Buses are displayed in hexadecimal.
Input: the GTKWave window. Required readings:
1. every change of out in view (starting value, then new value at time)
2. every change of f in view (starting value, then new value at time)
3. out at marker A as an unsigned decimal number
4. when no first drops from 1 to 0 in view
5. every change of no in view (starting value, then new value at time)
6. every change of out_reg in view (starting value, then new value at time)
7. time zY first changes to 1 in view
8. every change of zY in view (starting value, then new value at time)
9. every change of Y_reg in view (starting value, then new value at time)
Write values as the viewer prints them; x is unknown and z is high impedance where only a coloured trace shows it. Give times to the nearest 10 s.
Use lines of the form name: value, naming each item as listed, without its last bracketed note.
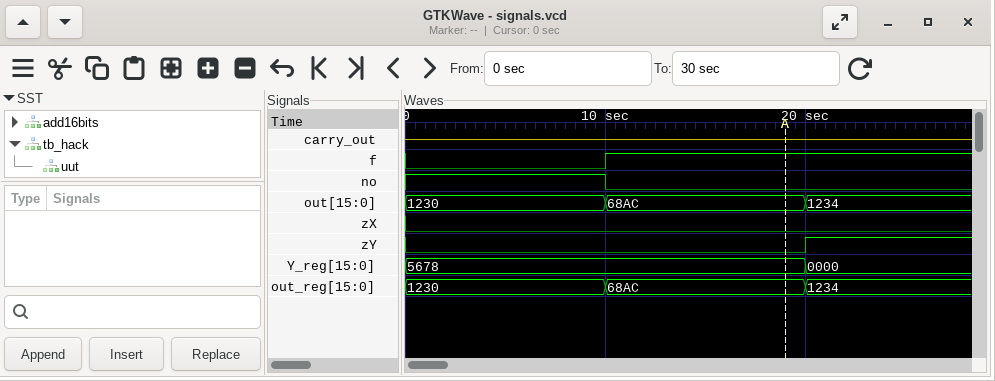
every change of out in view: 1230, 68AC at 10 s, 1234 at 20 s
every change of f in view: 0, 1 at 10 s
out at marker A as an unsigned decimal number: 26796
when no first drops from 1 to 0 in view: 10 s
every change of no in view: 1, 0 at 10 s
every change of out_reg in view: 1230, 68AC at 10 s, 1234 at 20 s
time zY first changes to 1 in view: 20 s
every change of zY in view: 0, 1 at 20 s
every change of Y_reg in view: 5678, 0000 at 20 s
